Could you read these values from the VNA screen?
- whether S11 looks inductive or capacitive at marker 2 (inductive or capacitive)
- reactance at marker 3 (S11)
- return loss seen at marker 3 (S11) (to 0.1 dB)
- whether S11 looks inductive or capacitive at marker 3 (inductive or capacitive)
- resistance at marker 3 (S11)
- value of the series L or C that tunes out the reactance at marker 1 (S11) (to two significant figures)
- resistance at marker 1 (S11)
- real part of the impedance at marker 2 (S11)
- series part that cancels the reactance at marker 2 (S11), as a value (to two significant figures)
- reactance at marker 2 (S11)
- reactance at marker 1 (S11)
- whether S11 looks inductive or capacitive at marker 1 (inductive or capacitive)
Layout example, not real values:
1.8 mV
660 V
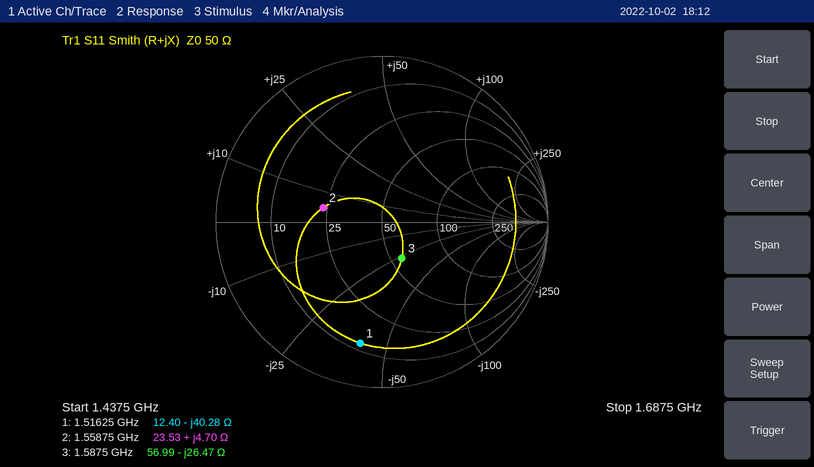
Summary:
inductive
-26.47 Ω
12.1 dB
capacitive
56.99 Ω
4.2 nH
12.40 Ω
23.53 Ω
22 pF
+4.70 Ω
-40.28 Ω
capacitive
